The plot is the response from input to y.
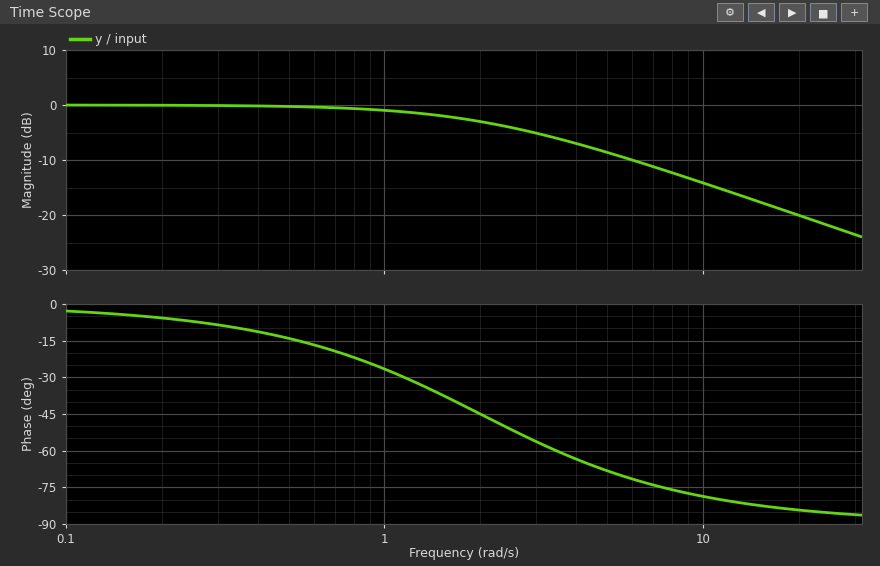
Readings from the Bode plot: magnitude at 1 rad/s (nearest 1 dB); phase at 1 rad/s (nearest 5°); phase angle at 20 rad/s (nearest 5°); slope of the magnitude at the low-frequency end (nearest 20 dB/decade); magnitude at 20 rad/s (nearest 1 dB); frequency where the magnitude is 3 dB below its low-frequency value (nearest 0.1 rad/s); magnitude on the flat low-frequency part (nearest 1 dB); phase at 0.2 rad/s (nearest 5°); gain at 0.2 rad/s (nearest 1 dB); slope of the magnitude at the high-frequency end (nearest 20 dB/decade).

-1 dB
-25°
-85°
0 dB/decade
-20 dB
2.0 rad/s
0 dB
-5°
0 dB
-20 dB/decade
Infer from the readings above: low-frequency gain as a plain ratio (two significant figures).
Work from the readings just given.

1.0
